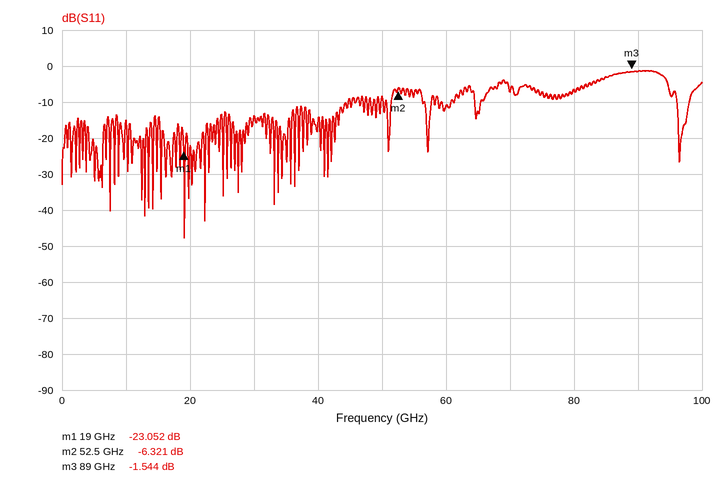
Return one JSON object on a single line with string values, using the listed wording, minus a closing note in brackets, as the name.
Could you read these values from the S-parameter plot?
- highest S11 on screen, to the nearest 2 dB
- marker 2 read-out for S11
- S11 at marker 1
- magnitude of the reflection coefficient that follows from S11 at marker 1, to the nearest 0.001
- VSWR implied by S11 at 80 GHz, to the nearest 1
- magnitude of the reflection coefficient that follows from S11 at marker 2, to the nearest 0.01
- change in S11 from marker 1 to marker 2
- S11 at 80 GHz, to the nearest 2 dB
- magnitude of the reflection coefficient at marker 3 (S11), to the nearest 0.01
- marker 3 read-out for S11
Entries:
{"highest S11 on screen, to the nearest 2 dB": "-2 dB", "marker 2 read-out for S11": "-6.321 dB", "S11 at marker 1": "-23.052 dB", "magnitude of the reflection coefficient that follows from S11 at marker 1, to the nearest 0.001": "0.070", "VSWR implied by S11 at 80 GHz, to the nearest 1": "3", "magnitude of the reflection coefficient that follows from S11 at marker 2, to the nearest 0.01": "0.48", "change in S11 from marker 1 to marker 2": "16.731 dB", "S11 at 80 GHz, to the nearest 2 dB": "-6 dB", "magnitude of the reflection coefficient at marker 3 (S11), to the nearest 0.01": "0.84", "marker 3 read-out for S11": "-1.544 dB"}
